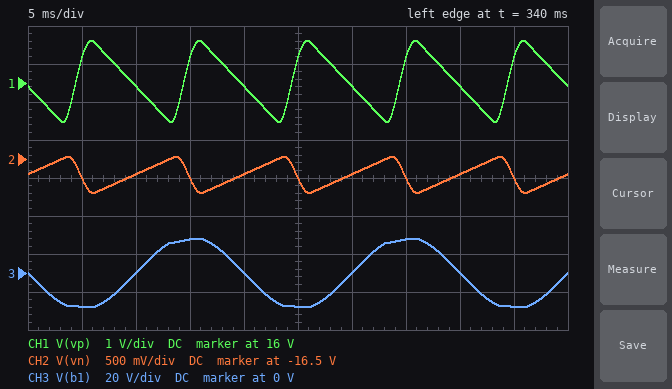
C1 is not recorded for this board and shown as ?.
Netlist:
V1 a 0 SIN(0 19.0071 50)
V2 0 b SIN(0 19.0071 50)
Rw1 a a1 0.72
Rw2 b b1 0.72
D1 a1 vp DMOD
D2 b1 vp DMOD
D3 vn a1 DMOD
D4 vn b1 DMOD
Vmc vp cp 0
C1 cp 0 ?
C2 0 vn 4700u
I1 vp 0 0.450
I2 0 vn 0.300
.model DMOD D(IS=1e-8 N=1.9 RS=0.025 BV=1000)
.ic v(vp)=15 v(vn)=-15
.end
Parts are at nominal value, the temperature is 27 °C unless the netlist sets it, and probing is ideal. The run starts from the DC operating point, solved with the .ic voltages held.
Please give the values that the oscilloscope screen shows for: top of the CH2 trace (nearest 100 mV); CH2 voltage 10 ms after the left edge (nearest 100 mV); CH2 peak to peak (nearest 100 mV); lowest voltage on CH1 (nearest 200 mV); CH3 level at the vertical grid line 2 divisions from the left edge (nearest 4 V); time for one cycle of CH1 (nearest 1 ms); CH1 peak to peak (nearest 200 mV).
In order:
-16.5 V
-16.7 V
500 mV
15.0 V
0 V
10 ms
2.2 V
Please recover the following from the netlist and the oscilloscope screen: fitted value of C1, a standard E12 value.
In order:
1.5 mF
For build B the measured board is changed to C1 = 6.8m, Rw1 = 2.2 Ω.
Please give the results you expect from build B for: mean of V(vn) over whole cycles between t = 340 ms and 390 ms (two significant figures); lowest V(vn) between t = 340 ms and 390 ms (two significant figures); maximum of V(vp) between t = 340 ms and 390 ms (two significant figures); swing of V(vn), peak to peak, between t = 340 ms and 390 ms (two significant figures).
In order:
-16 V
-17 V
16 V
760 mV
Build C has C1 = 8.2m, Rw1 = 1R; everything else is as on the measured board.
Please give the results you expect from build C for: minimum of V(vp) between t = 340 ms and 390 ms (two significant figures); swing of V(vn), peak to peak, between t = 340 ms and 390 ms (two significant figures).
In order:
16 V
570 mV
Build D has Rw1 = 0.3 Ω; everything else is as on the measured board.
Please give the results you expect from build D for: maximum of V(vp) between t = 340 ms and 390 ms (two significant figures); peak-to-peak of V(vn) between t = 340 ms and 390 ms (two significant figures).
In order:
18 V
720 mV
